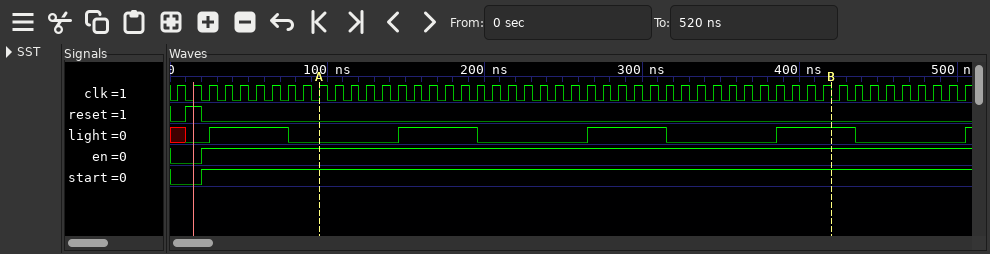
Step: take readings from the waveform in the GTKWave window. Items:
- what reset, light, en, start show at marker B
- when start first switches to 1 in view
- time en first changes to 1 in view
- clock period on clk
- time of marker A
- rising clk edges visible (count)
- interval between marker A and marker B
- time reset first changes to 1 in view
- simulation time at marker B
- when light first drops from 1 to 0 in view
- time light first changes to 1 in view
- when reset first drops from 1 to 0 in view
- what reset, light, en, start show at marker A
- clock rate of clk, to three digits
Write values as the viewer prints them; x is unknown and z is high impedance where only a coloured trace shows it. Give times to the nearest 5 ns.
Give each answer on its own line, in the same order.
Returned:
reset=0, light=1, en=1, start=1
20 ns
20 ns
10 ns
95 ns
51
325 ns
10 ns
420 ns
75 ns
25 ns
20 ns
reset=0, light=0, en=1, start=1
100 MHz
